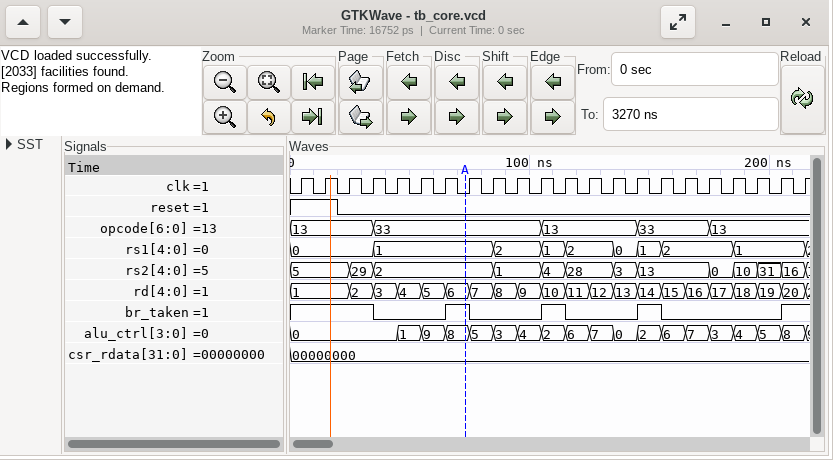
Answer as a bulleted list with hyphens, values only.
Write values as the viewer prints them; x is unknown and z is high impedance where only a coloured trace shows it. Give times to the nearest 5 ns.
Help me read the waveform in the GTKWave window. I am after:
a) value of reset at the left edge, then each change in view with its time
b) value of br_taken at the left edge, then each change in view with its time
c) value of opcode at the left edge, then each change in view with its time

- 1, 0 at 20 ns
- 1, 0 at 35 ns, 1 at 65 ns, 0 at 75 ns, 1 at 105 ns, 0 at 115 ns, 1 at 145 ns, 0 at 155 ns, 1 at 205 ns
- 13, 33 at 35 ns, 13 at 105 ns, 33 at 145 ns, 13 at 175 ns
